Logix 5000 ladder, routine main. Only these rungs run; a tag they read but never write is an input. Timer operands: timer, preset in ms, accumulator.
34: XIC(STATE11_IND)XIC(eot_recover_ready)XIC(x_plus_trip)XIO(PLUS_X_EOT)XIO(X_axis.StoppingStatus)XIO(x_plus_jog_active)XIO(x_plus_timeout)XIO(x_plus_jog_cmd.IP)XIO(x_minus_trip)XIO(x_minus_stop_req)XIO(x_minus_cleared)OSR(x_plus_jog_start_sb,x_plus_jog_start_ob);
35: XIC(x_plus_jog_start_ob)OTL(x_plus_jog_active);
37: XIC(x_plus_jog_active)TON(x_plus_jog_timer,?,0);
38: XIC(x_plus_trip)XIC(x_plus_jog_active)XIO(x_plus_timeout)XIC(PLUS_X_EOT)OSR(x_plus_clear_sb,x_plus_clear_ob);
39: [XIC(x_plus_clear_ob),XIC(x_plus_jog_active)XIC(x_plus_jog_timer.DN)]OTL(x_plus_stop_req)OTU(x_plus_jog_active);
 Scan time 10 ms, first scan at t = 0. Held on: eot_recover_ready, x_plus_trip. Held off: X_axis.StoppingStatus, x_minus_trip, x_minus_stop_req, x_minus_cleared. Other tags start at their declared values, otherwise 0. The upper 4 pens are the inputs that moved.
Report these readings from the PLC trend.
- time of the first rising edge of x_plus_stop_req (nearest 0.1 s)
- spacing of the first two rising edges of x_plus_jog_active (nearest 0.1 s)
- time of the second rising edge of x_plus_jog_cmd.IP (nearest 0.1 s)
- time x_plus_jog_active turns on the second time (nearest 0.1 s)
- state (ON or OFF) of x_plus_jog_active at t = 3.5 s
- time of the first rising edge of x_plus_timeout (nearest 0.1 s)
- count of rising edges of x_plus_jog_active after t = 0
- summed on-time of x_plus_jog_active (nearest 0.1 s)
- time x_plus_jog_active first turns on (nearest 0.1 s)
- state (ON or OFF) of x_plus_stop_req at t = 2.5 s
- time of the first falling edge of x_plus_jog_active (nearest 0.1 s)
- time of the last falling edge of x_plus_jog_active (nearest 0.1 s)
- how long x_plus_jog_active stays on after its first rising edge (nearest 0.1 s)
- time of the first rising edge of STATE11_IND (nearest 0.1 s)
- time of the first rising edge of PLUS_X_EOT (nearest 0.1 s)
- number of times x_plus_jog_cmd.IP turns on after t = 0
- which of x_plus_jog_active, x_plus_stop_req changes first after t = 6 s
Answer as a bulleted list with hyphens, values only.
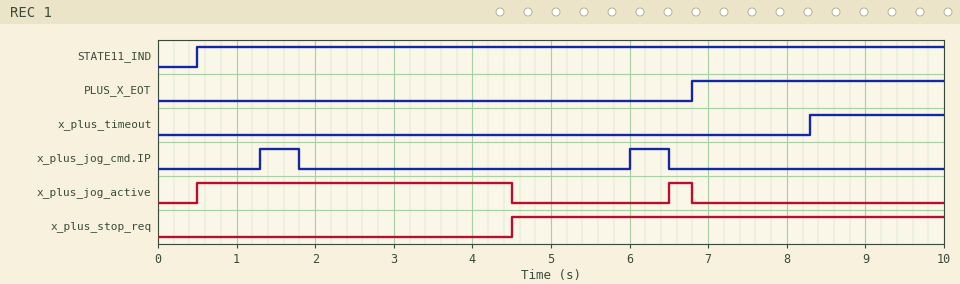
- 4.5 s
- 6.0 s
- 6.0 s
- 6.5 s
- ON
- 8.3 s
- 2
- 4.3 s
- 0.5 s
- OFF
- 4.5 s
- 6.8 s
- 4.0 s
- 0.5 s
- 6.8 s
- 2
- x_plus_jog_active
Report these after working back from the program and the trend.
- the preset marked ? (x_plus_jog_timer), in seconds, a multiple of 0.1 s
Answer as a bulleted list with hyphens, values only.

- 4.0 s
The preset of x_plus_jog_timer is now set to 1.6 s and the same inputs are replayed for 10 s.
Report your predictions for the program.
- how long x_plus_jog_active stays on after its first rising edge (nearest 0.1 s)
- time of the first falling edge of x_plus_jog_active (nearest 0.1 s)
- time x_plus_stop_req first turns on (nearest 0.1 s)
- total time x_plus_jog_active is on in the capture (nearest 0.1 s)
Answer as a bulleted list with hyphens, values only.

- 1.6 s
- 2.1 s
- 2.1 s
- 1.9 s
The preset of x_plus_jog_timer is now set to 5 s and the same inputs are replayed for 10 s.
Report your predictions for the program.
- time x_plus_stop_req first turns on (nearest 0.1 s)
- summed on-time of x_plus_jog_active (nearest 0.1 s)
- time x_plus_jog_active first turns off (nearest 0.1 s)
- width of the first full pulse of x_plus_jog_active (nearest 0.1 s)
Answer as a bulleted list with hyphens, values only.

- 5.5 s
- 5.3 s
- 5.5 s
- 5.0 s
